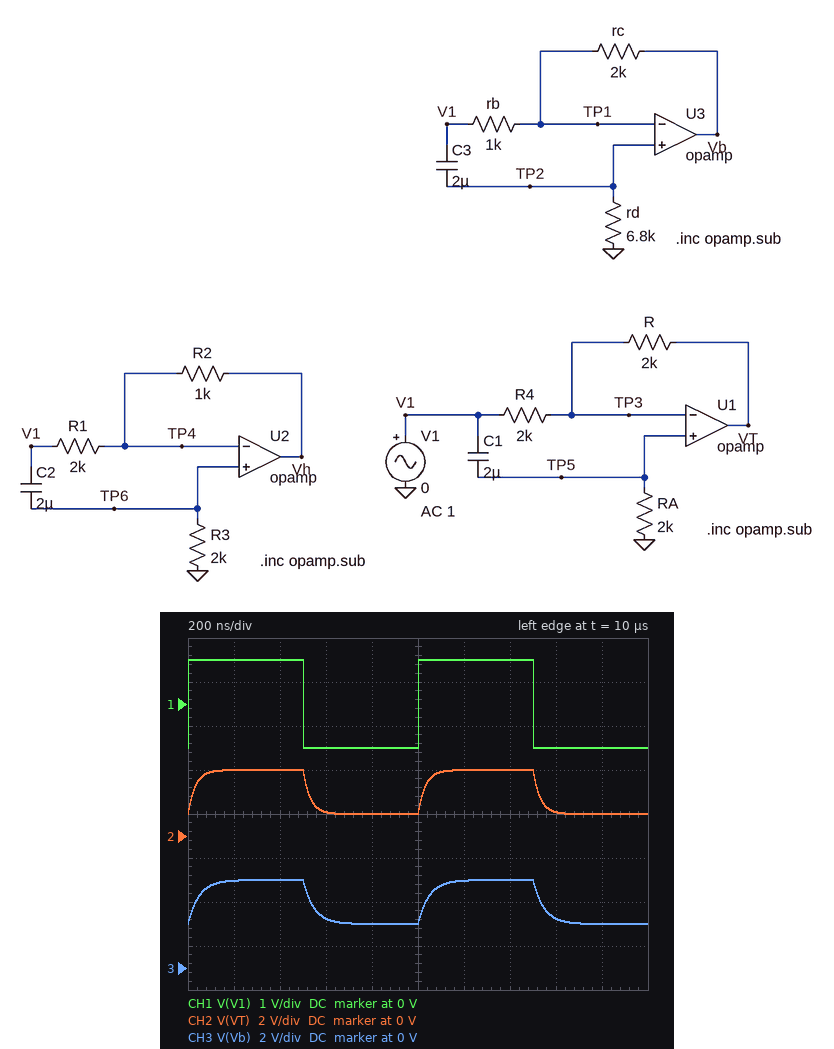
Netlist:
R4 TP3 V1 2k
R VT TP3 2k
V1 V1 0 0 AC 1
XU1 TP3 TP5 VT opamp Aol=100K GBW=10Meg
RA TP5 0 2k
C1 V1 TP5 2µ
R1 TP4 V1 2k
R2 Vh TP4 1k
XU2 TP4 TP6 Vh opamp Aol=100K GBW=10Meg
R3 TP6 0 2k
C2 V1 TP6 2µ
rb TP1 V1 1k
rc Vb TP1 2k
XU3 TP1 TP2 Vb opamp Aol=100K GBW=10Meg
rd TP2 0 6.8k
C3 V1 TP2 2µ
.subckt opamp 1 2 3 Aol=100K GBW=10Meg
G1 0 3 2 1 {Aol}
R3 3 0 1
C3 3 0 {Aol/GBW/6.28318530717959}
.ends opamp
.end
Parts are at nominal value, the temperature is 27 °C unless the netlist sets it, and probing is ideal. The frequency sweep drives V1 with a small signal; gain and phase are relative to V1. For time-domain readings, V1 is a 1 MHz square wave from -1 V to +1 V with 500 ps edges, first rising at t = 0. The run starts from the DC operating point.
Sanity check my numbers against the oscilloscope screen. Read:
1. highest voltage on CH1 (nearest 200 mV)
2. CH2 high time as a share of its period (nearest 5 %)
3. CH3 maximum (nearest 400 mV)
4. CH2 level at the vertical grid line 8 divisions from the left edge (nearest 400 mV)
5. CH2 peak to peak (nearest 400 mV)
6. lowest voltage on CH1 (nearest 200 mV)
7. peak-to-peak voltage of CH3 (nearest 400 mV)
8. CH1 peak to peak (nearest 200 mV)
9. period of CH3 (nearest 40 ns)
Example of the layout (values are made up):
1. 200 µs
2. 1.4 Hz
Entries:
1. 1.0 V
2. 50 %
3. 4.0 V
4. 1.2 V
5. 2.0 V
6. -1.0 V
7. 2.0 V
8. 2.0 V
9. 1.00 µs
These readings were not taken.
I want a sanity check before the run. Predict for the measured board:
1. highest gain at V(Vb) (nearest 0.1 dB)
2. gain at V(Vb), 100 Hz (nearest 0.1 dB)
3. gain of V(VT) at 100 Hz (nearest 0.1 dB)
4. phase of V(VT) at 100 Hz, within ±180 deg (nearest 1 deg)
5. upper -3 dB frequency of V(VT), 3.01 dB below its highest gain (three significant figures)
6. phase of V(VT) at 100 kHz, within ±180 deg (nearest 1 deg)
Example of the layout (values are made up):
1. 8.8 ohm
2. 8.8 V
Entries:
1. 6.0 dB
2. 0.2 dB
3. 0 dB
4. 43 deg
5. 5.00 MHz
6. -1 deg
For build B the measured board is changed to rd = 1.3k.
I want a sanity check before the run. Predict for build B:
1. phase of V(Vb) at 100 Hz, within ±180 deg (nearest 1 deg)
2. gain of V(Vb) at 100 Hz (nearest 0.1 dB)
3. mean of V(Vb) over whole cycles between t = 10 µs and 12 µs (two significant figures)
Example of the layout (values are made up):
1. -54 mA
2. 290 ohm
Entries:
1. 82 deg
2. 2.6 dB
3. 3.0 V
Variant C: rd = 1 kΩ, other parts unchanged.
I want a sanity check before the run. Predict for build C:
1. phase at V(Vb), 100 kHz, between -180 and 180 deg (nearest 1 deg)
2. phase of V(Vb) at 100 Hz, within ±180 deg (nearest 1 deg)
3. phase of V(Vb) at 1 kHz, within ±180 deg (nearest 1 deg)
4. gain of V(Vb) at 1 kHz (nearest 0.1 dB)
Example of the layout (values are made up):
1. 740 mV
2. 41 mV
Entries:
1. -2 deg
2. 96 deg
3. 14 deg
4. 0.1 dB
